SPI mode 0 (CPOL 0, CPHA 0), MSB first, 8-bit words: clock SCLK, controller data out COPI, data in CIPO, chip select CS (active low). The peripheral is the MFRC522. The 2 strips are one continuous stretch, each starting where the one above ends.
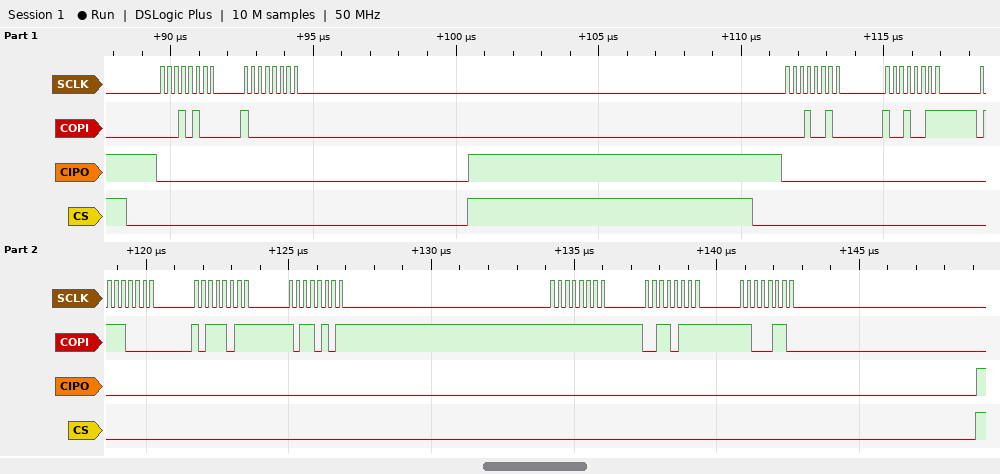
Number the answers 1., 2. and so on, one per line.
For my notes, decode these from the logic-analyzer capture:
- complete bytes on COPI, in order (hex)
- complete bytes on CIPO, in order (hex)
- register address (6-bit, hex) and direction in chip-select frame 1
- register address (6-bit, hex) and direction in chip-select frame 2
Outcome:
1. 14 80 12 93 70 BB B5 FF 37 C6
2. 00 00 00 00 00 00 00 00 00 00
3. 0x0A write
4. 0x09 write
